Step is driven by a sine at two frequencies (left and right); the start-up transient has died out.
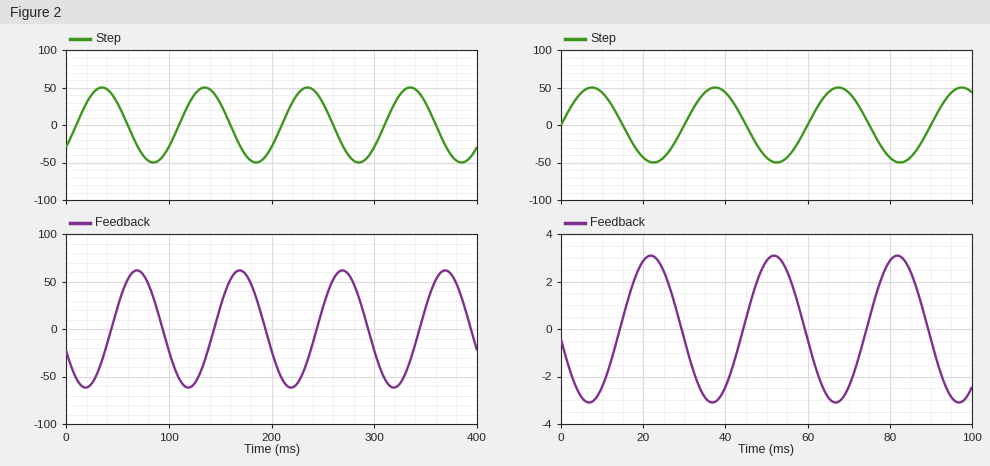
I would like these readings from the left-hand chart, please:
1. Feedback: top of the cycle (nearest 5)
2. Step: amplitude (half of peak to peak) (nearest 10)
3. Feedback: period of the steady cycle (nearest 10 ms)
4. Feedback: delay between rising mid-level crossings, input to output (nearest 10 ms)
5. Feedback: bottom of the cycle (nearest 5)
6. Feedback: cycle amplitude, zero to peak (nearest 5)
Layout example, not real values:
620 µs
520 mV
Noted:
60
50
100 ms
30 ms
-60
60
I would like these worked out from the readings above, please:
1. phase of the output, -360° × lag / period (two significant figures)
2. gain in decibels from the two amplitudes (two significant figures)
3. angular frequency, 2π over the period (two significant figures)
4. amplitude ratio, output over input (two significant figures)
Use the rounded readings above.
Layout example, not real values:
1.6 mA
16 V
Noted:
-110°
1.6 dB
0.063 rad/ms
1.2
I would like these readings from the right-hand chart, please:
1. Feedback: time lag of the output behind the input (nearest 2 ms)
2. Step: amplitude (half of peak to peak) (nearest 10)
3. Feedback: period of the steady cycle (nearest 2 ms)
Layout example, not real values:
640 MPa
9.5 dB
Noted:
14 ms
50
30 ms
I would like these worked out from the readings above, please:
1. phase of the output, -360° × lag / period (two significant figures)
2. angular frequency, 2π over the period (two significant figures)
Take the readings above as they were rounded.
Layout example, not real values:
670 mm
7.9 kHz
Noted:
-170°
0.21 rad/ms
